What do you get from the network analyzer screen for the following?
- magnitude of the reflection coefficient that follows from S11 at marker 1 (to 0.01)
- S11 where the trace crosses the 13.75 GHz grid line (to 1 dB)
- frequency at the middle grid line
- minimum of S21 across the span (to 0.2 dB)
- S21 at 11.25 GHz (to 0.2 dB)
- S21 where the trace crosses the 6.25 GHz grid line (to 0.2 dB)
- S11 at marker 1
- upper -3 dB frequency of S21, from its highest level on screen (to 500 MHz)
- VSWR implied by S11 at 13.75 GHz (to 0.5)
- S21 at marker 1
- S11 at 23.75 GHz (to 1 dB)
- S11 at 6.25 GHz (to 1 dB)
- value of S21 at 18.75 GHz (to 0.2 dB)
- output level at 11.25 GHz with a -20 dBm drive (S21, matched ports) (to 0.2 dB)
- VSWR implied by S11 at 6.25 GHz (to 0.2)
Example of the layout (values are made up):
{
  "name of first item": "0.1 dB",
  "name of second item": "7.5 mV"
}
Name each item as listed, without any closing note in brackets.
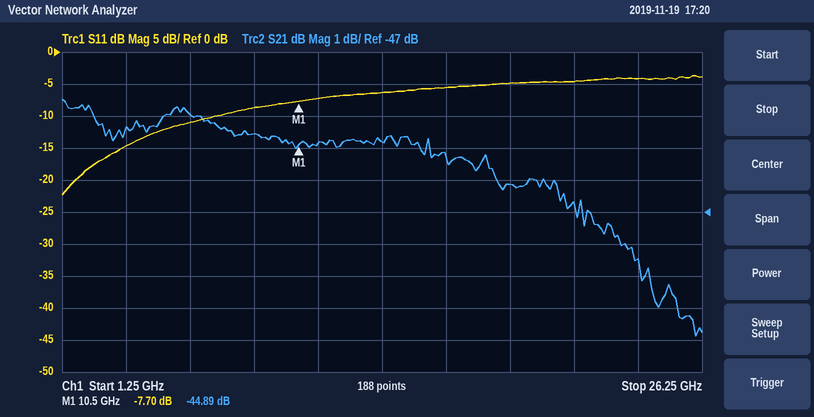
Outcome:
{
  "magnitude of the reflection coefficient that follows from S11 at marker 1": "0.41",
  "S11 where the trace crosses the 13.75 GHz grid line": "-6 dB",
  "frequency at the middle grid line": "13.75 GHz",
  "minimum of S21 across the span": "-50.8 dB",
  "S21 at 11.25 GHz": "-44.8 dB",
  "S21 where the trace crosses the 6.25 GHz grid line": "-44.0 dB",
  "S11 at marker 1": "-7.70 dB",
  "upper -3 dB frequency of S21, from its highest level on screen": "20.5 GHz",
  "VSWR implied by S11 at 13.75 GHz": "3.0",
  "S21 at marker 1": "-44.89 dB",
  "S11 at 23.75 GHz": "-4 dB",
  "S11 at 6.25 GHz": "-11 dB",
  "value of S21 at 18.75 GHz": "-46.2 dB",
  "output level at 11.25 GHz with a -20 dBm drive (S21, matched ports)": "-64.8 dBm",
  "VSWR implied by S11 at 6.25 GHz": "1.8"
}
